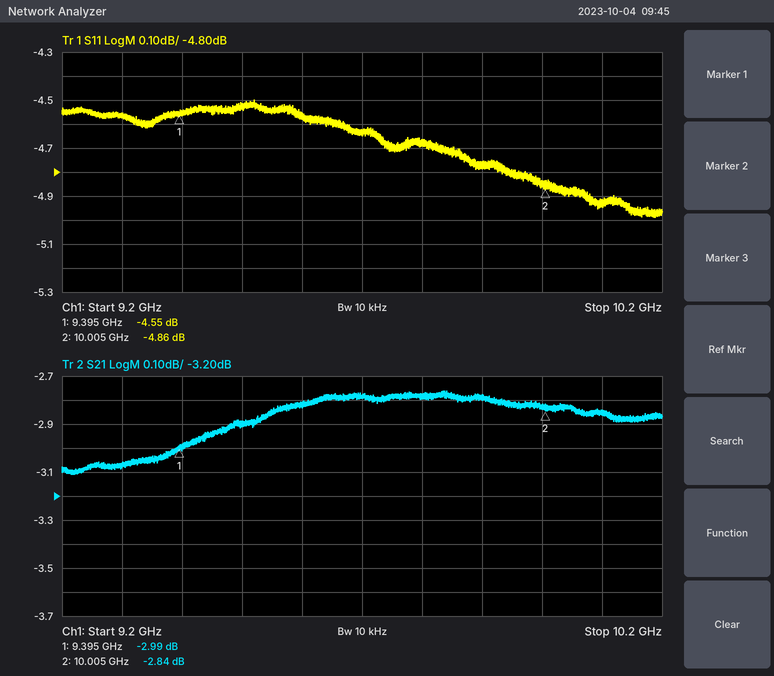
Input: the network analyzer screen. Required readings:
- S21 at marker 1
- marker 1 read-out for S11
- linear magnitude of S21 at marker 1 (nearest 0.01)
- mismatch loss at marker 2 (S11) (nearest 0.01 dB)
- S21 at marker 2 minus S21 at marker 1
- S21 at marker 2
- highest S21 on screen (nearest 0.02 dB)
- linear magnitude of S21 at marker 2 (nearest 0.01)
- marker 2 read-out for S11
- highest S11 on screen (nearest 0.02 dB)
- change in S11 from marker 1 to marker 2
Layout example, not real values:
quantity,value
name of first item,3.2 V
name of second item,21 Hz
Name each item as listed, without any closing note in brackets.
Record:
quantity,value
S21 at marker 1,-2.99 dB
marker 1 read-out for S11,-4.55 dB
linear magnitude of S21 at marker 1,0.71
mismatch loss at marker 2 (S11),1.72 dB
S21 at marker 2 minus S21 at marker 1,0.15 dB
S21 at marker 2,-2.84 dB
highest S21 on screen,-2.76 dB
linear magnitude of S21 at marker 2,0.72
marker 2 read-out for S11,-4.86 dB
highest S11 on screen,-4.50 dB
change in S11 from marker 1 to marker 2,-0.31 dB
